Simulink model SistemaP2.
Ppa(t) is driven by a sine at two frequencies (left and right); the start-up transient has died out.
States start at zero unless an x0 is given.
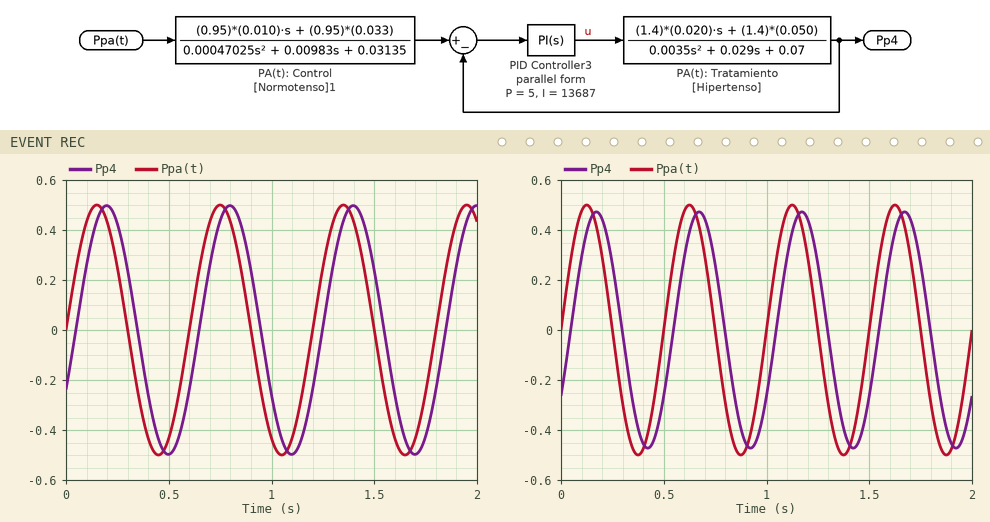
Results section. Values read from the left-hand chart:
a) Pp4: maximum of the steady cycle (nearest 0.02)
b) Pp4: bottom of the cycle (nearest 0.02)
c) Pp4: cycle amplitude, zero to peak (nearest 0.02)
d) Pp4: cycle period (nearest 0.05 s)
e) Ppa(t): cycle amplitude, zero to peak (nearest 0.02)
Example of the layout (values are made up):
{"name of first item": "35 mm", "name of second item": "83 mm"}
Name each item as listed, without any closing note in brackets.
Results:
{"Pp4: maximum of the steady cycle": "0.50", "Pp4: bottom of the cycle": "-0.50", "Pp4: cycle amplitude, zero to peak": "0.50", "Pp4: cycle period": "0.60 s", "Ppa(t): cycle amplitude, zero to peak": "0.50"}
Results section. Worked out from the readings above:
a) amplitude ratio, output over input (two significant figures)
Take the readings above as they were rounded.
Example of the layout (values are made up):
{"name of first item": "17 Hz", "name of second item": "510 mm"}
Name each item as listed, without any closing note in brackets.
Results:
{"amplitude ratio, output over input": "1.0"}
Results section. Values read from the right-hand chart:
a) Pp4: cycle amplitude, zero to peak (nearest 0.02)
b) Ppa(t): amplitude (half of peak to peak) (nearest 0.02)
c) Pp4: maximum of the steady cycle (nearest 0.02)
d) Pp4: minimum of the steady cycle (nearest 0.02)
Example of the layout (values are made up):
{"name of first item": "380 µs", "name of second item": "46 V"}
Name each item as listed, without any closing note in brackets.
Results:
{"Pp4: cycle amplitude, zero to peak": "0.48", "Ppa(t): amplitude (half of peak to peak)": "0.50", "Pp4: maximum of the steady cycle": "0.48", "Pp4: minimum of the steady cycle": "-0.48"}
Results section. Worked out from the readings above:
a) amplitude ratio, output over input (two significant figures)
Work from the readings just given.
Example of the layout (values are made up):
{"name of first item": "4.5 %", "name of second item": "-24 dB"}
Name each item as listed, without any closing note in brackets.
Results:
{"amplitude ratio, output over input": "0.96"}
